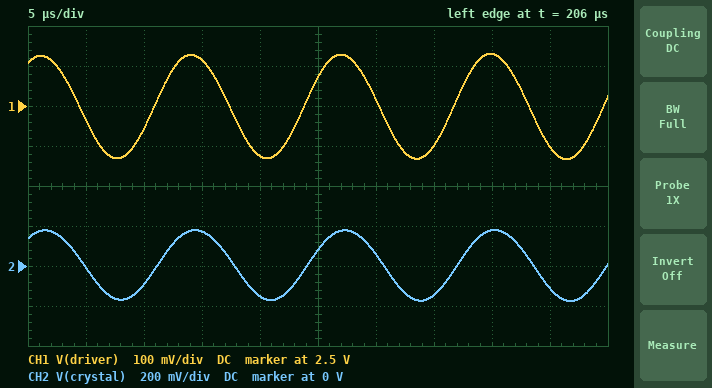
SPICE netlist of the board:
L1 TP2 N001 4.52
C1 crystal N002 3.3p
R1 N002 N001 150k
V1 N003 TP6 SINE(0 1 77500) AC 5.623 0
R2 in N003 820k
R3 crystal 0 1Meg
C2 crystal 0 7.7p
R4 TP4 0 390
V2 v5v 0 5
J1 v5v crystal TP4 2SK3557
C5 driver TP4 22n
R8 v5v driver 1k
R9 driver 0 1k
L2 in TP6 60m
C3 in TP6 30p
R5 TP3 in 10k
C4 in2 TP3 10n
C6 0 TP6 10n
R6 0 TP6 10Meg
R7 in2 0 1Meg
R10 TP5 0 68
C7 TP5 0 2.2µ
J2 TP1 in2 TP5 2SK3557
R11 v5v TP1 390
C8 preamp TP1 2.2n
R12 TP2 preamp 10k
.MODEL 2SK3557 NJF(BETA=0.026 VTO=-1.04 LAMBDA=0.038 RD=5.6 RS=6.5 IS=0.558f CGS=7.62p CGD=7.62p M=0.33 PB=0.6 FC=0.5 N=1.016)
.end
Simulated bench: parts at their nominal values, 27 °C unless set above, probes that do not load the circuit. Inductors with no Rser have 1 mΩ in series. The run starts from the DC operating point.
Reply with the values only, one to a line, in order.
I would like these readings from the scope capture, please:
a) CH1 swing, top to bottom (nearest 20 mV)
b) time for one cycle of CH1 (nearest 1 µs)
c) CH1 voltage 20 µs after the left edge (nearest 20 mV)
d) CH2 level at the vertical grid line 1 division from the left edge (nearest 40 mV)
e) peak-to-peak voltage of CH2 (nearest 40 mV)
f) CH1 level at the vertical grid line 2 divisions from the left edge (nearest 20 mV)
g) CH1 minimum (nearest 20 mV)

260 mV
13 µs
2.38 V
0 V
360 mV
2.44 V
2.36 V
